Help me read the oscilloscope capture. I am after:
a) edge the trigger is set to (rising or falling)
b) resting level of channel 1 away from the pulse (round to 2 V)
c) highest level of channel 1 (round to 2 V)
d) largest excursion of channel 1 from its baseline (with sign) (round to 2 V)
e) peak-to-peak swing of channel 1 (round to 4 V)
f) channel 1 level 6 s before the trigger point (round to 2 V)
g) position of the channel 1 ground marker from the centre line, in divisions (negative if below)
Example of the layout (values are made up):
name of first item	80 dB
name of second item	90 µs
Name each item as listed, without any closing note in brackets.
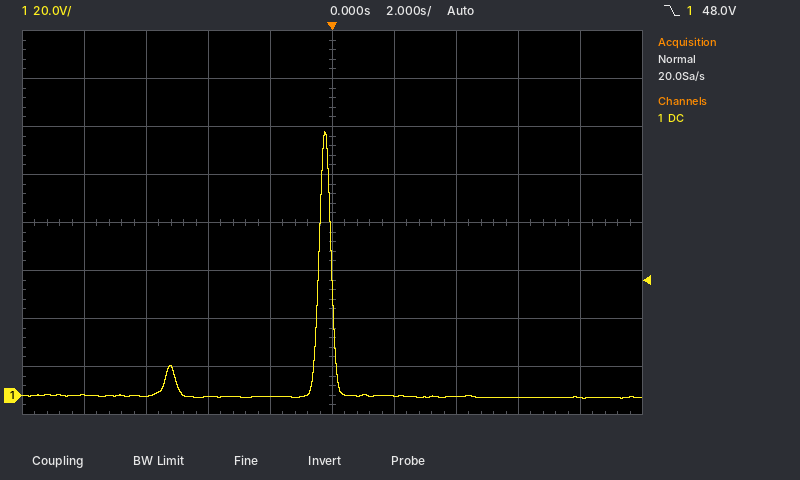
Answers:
edge the trigger is set to	falling
resting level of channel 1 away from the pulse	0 V
highest level of channel 1	110 V
largest excursion of channel 1 from its baseline (with sign)	+110 V
peak-to-peak swing of channel 1	112 V
channel 1 level 6 s before the trigger point	0 V
position of the channel 1 ground marker from the centre line, in divisions	-3.6 div
